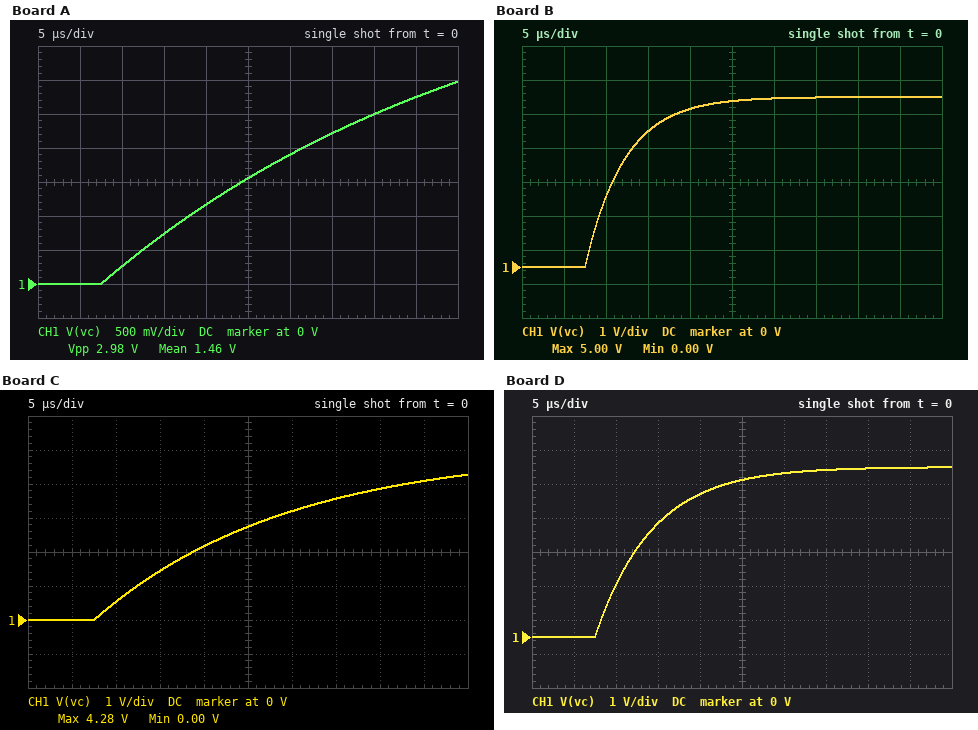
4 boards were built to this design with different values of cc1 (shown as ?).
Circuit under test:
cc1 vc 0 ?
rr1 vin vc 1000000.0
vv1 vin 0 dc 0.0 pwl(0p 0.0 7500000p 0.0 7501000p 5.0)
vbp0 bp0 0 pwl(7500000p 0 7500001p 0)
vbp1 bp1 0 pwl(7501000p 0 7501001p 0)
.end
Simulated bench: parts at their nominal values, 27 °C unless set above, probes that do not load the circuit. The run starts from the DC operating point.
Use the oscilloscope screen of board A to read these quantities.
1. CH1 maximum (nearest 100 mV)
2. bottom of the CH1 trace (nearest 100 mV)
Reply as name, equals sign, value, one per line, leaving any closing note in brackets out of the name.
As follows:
CH1 maximum = 3.0 V
bottom of the CH1 trace = 0 V
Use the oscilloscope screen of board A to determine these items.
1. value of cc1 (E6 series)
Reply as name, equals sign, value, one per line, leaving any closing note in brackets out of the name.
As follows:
value of cc1 = 47 pF
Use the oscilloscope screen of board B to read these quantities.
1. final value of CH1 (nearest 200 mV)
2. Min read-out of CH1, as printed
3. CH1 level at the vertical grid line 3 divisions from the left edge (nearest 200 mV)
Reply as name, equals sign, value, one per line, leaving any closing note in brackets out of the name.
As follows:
final value of CH1 = 5.0 V
Min read-out of CH1, as printed = 0.00 V
CH1 level at the vertical grid line 3 divisions from the left edge = 4.0 V
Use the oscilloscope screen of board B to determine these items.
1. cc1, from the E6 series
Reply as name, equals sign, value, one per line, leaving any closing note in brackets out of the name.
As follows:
cc1, from the E6 series = 4.7 pF
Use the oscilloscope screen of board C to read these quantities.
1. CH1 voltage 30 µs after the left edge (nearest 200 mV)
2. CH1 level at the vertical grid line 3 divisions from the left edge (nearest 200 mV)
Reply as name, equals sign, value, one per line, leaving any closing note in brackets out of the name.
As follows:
CH1 voltage 30 µs after the left edge = 3.2 V
CH1 level at the vertical grid line 3 divisions from the left edge = 1.4 V
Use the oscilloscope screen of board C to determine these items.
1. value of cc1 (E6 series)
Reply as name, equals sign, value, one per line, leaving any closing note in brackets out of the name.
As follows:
value of cc1 = 22 pF
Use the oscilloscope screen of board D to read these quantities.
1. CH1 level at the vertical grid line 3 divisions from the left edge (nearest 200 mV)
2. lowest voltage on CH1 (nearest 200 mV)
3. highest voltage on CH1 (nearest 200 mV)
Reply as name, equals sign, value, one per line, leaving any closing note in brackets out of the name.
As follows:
CH1 level at the vertical grid line 3 divisions from the left edge = 3.4 V
lowest voltage on CH1 = 0 V
highest voltage on CH1 = 5.0 V
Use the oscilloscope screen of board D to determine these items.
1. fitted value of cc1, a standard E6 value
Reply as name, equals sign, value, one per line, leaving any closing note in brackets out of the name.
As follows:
fitted value of cc1, a standard E6 value = 6.8 pF
